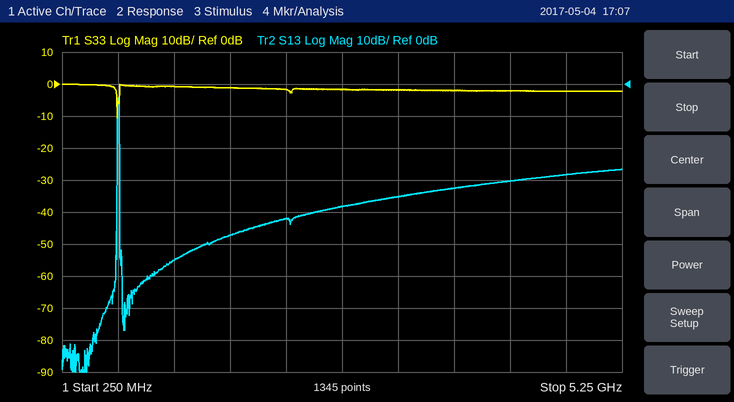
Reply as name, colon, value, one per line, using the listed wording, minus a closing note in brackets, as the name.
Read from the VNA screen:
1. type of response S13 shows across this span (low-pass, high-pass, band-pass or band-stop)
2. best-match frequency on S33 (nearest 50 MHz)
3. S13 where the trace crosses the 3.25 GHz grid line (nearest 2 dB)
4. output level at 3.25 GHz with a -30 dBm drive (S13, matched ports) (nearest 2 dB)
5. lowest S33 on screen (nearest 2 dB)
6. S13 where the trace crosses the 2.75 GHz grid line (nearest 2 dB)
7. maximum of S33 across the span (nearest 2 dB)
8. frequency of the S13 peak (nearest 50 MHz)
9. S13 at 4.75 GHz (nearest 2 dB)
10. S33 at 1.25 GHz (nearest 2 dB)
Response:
type of response S13 shows across this span: band-pass
best-match frequency on S33: 750 MHz
S13 where the trace crosses the 3.25 GHz grid line: -36 dB
output level at 3.25 GHz with a -30 dBm drive (S13, matched ports): -66 dBm
lowest S33 on screen: -10 dB
S13 where the trace crosses the 2.75 GHz grid line: -38 dB
maximum of S33 across the span: 0 dB
frequency of the S13 peak: 750 MHz
S13 at 4.75 GHz: -28 dB
S33 at 1.25 GHz: 0 dB
